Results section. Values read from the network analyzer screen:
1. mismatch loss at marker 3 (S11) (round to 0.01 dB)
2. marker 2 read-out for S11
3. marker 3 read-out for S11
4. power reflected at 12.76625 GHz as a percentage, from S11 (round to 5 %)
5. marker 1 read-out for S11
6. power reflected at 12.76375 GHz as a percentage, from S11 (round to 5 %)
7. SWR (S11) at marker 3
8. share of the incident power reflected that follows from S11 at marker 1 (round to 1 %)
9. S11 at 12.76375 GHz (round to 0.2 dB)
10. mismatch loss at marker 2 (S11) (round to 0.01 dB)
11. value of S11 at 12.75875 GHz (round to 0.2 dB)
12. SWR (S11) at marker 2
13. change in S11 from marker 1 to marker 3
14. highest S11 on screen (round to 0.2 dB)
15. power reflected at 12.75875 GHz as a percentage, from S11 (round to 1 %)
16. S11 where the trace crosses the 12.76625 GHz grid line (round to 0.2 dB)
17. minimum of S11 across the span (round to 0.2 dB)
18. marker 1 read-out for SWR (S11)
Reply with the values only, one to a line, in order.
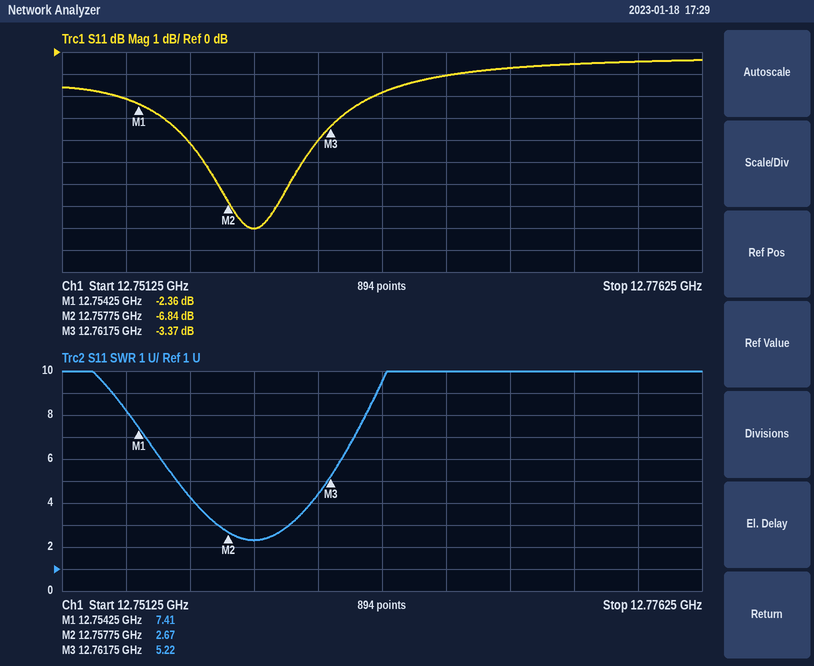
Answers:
2.68 dB
-6.84 dB
-3.37 dB
80 %
-2.36 dB
65 %
5.22
58 %
-1.8 dB
1.01 dB
-8.0 dB
2.67
-1.01 dB
-0.4 dB
16 %
-1.0 dB
-8.0 dB
7.41
